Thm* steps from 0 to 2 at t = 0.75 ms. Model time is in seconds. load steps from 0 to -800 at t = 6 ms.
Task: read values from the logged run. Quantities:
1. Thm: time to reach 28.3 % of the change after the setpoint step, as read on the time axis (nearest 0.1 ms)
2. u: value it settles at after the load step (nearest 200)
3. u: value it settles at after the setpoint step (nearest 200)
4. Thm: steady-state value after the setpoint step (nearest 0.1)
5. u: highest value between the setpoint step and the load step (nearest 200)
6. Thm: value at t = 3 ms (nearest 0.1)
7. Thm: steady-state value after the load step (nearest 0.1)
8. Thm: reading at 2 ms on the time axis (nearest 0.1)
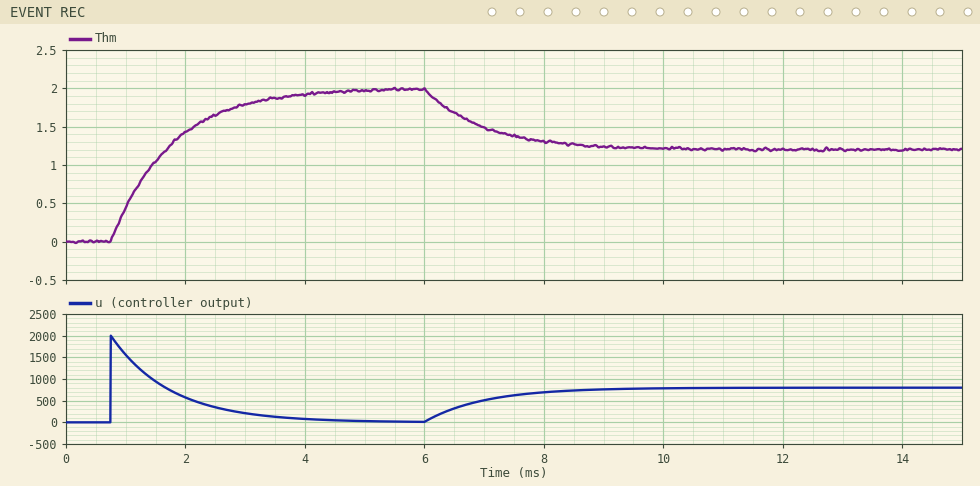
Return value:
1.1 ms
800
0
2.0
2000
1.8
1.2
1.4
